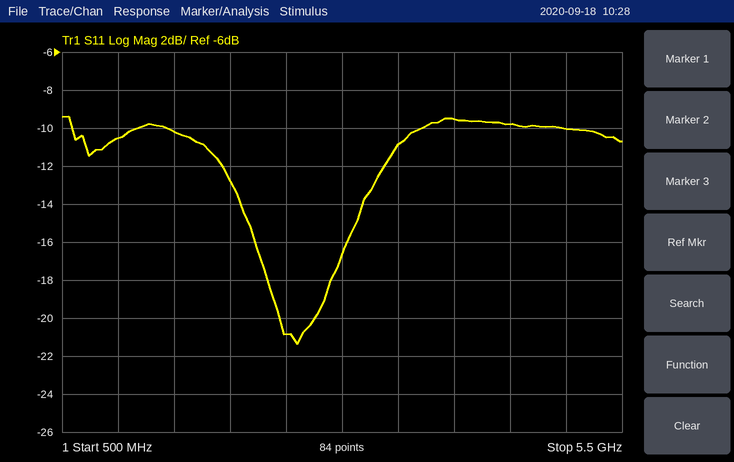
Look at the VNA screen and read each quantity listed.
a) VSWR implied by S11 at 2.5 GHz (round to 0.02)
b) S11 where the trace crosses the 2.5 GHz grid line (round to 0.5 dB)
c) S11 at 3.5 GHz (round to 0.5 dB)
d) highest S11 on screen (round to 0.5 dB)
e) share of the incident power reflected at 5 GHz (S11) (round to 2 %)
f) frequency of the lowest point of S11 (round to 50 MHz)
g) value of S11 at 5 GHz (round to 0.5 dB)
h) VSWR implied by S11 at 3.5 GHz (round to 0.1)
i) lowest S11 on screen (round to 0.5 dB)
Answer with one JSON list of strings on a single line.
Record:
["1.20", "-21.0 dB", "-11.0 dB", "-9.5 dB", "10 %", "2.60 GHz", "-10.0 dB", "1.8", "-21.5 dB"]
